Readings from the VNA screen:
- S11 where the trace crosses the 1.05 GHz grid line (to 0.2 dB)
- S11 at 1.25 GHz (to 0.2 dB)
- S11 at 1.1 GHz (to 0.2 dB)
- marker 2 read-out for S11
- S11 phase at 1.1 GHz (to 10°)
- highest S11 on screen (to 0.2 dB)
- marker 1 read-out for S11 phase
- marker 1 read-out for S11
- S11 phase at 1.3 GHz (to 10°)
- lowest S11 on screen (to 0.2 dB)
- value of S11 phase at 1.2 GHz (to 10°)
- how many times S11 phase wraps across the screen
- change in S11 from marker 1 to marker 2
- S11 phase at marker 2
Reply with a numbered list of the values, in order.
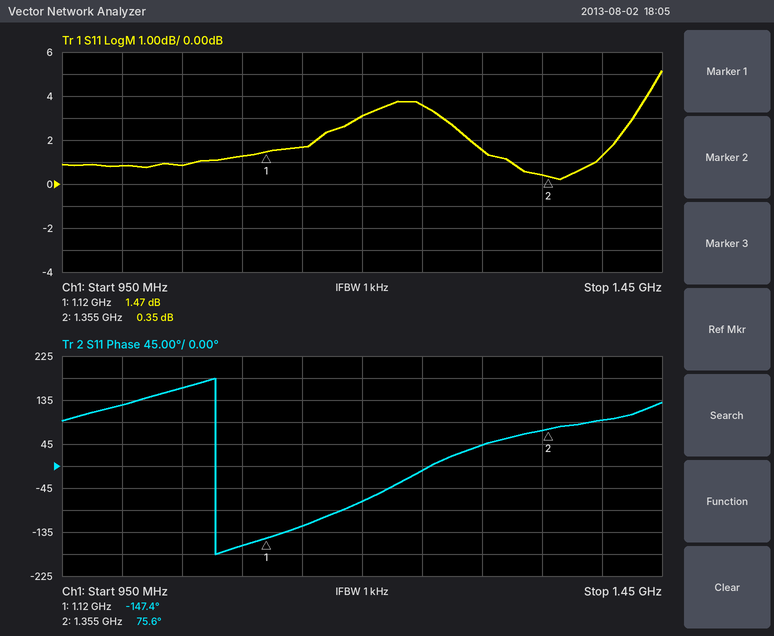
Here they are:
1. 0.8 dB
2. 3.6 dB
3. 1.2 dB
4. 0.35 dB
5. -160°
6. 5.2 dB
7. -147.4°
8. 1.47 dB
9. 40°
10. 0.2 dB
11. -70°
12. 1
13. -1.12 dB
14. 75.6°
